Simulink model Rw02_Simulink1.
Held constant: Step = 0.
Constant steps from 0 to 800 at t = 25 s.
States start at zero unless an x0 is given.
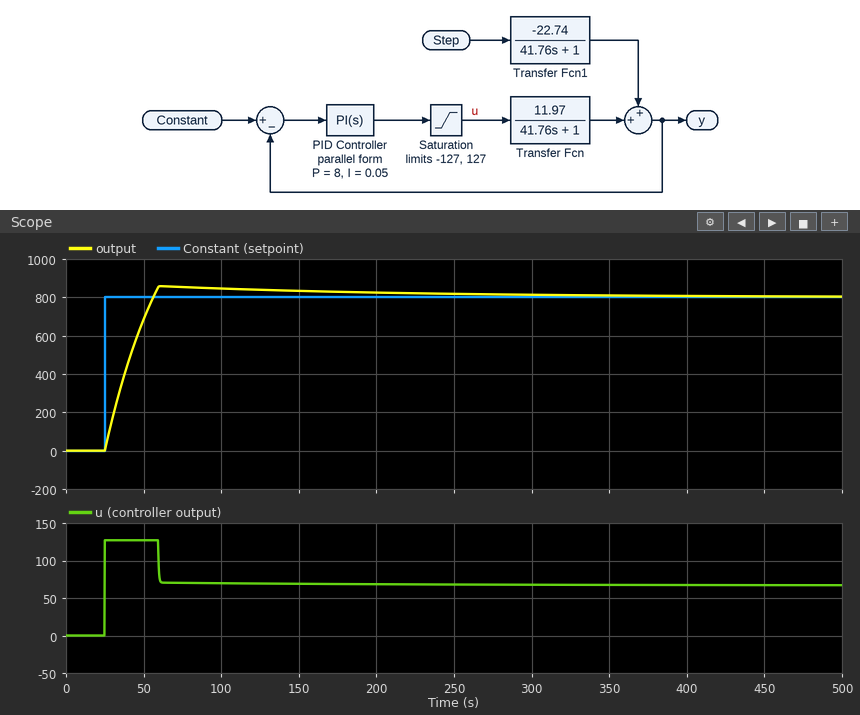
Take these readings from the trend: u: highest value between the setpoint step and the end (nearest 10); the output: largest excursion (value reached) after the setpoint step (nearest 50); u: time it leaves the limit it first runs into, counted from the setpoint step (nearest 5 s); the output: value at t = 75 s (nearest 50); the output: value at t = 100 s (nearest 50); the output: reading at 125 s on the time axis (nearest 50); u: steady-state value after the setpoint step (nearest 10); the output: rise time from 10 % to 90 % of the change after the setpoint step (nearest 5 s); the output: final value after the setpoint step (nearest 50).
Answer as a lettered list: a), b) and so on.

a) 130
b) 850
c) 35 s
d) 850
e) 850
f) 850
g) 70
h) 25 s
i) 800
